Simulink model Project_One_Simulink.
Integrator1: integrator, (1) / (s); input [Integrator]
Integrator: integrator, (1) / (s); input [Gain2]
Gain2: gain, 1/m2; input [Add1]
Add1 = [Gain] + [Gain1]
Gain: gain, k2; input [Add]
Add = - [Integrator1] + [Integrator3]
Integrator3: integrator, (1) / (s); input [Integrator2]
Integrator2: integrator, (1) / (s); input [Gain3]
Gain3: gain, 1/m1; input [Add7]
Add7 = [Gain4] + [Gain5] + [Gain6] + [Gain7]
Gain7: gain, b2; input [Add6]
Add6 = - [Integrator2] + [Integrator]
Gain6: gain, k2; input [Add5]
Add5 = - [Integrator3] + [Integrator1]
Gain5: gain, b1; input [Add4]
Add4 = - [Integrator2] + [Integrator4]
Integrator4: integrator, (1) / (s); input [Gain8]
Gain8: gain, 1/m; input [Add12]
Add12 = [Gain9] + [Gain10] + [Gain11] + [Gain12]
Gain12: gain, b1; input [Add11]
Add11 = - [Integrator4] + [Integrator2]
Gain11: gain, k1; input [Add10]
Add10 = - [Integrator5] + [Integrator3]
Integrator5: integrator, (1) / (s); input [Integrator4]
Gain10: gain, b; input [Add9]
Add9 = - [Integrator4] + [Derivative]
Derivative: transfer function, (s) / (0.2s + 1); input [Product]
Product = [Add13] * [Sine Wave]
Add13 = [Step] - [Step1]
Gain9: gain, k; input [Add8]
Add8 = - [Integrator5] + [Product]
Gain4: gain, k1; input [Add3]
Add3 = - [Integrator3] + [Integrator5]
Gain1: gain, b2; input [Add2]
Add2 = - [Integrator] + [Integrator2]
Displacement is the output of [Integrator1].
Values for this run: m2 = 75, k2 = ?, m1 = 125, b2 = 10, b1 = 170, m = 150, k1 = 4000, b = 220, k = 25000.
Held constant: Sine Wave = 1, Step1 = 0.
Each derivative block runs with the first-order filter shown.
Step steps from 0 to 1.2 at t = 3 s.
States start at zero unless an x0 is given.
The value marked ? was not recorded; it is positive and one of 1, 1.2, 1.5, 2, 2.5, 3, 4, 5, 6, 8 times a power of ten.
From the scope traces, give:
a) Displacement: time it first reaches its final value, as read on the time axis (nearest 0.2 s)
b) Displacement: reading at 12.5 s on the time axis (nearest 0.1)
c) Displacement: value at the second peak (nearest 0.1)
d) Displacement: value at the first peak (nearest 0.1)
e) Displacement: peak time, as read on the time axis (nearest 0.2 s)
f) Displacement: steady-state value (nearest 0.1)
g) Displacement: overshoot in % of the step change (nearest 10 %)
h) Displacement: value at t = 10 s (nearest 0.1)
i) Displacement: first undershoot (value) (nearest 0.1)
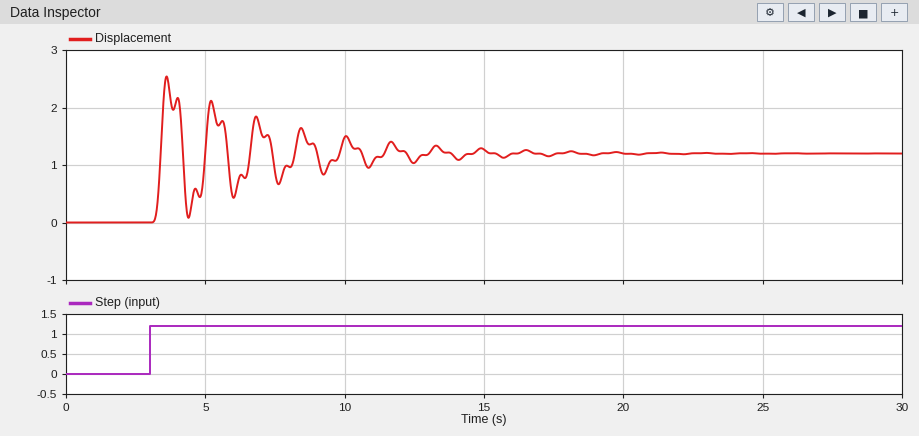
3.4 s
1.0
2.2
2.5
3.6 s
1.2
110 %
1.5
2.0
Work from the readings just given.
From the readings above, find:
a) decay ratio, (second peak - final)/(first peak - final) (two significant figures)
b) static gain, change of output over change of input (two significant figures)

0.77
1.0
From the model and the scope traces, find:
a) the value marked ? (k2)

6000
